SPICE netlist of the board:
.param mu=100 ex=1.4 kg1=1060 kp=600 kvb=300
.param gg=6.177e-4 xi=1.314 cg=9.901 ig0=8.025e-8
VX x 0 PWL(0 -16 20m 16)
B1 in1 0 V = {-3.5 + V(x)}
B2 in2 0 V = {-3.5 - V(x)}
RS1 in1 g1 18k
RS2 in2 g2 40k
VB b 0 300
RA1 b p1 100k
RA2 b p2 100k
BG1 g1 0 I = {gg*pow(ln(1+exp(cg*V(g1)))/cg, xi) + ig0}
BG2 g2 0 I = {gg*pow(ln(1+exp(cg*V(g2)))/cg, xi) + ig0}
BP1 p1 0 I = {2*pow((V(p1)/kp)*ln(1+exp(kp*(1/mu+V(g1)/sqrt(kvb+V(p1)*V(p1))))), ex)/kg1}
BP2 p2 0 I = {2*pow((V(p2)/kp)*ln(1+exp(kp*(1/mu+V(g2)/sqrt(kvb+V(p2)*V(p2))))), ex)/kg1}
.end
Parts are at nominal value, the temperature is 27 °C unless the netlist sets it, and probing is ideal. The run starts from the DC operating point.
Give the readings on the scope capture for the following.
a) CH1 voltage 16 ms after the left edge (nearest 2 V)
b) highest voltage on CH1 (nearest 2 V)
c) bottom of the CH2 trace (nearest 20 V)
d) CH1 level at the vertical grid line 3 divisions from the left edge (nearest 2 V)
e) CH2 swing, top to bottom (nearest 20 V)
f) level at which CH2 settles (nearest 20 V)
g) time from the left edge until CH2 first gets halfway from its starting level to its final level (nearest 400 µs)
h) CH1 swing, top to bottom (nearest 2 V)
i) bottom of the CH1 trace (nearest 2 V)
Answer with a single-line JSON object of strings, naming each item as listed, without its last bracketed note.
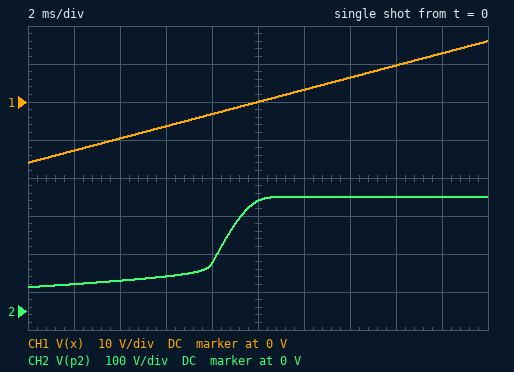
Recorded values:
{"CH1 voltage 16 ms after the left edge": "10 V", "highest voltage on CH1": "16 V", "bottom of the CH2 trace": "60 V", "CH1 level at the vertical grid line 3 divisions from the left edge": "-6 V", "CH2 swing, top to bottom": "240 V", "level at which CH2 settles": "300 V", "time from the left edge until CH2 first gets halfway from its starting level to its final level": "8.4 ms", "CH1 swing, top to bottom": "32 V", "bottom of the CH1 trace": "-16 V"}
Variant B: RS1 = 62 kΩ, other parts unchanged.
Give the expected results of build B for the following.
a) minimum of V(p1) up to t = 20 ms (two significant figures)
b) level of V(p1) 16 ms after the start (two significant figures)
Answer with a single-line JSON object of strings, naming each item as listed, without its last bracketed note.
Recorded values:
{"minimum of V(p1) up to t = 20 ms": "74 V", "level of V(p1) 16 ms after the start": "87 V"}
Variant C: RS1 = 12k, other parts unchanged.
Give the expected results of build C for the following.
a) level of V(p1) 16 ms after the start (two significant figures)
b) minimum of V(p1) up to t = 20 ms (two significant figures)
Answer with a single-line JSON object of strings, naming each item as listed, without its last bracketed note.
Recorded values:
{"level of V(p1) 16 ms after the start": "50 V", "minimum of V(p1) up to t = 20 ms": "46 V"}
